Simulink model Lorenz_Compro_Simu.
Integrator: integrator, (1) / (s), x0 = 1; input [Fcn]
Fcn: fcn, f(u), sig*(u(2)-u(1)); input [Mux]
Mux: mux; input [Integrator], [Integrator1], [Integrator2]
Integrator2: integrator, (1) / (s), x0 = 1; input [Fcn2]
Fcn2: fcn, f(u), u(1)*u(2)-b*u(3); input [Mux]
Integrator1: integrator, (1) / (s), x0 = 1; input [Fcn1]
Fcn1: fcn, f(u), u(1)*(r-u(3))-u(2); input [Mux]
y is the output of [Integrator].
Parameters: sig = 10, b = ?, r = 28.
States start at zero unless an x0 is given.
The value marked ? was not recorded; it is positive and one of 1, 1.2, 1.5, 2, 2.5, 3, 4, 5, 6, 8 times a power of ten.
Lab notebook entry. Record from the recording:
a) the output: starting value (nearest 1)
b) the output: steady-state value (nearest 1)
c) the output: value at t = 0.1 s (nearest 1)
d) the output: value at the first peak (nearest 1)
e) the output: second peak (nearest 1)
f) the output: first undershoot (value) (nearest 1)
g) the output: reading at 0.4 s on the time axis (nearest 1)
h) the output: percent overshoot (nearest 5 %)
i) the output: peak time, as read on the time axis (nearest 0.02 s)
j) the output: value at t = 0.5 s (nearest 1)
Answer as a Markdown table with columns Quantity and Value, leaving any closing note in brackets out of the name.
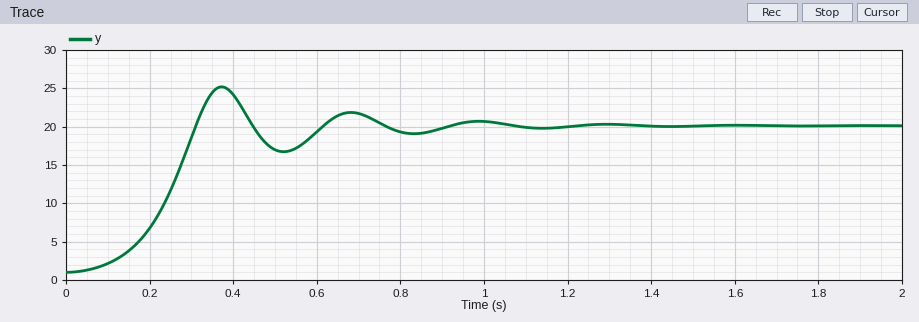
| Quantity | Value |
|---|---|
| the output: starting value | 1 |
| the output: steady-state value | 20 |
| the output: value at t = 0.1 s | 2 |
| the output: value at the first peak | 25 |
| the output: second peak | 22 |
| the output: first undershoot (value) | 17 |
| the output: reading at 0.4 s on the time axis | 24 |
| the output: percent overshoot | 25 % |
| the output: peak time, as read on the time axis | 0.38 s |
| the output: value at t = 0.5 s | 17 |
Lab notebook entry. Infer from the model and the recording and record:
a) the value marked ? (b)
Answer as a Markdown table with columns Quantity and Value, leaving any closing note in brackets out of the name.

| Quantity | Value |
|---|---|
| the value marked ? | 15 |
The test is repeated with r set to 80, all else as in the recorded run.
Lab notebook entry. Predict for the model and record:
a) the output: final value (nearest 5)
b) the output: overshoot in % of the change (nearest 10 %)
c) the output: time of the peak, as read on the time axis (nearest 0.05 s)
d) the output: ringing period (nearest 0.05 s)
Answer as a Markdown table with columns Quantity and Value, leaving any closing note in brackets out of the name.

| Quantity | Value |
|---|---|
| the output: final value | 35 |
| the output: overshoot in % of the change | 40 % |
| the output: time of the peak, as read on the time axis | 0.20 s |
| the output: ringing period | 0.20 s |
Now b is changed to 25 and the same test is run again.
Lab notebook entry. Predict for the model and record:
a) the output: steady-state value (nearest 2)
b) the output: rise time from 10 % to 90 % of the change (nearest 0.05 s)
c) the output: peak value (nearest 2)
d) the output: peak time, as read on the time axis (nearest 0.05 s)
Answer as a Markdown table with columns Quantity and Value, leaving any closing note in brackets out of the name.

| Quantity | Value |
|---|---|
| the output: steady-state value | 26 |
| the output: rise time from 10 % to 90 % of the change | 0.20 s |
| the output: peak value | 30 |
| the output: peak time, as read on the time axis | 0.40 s |
